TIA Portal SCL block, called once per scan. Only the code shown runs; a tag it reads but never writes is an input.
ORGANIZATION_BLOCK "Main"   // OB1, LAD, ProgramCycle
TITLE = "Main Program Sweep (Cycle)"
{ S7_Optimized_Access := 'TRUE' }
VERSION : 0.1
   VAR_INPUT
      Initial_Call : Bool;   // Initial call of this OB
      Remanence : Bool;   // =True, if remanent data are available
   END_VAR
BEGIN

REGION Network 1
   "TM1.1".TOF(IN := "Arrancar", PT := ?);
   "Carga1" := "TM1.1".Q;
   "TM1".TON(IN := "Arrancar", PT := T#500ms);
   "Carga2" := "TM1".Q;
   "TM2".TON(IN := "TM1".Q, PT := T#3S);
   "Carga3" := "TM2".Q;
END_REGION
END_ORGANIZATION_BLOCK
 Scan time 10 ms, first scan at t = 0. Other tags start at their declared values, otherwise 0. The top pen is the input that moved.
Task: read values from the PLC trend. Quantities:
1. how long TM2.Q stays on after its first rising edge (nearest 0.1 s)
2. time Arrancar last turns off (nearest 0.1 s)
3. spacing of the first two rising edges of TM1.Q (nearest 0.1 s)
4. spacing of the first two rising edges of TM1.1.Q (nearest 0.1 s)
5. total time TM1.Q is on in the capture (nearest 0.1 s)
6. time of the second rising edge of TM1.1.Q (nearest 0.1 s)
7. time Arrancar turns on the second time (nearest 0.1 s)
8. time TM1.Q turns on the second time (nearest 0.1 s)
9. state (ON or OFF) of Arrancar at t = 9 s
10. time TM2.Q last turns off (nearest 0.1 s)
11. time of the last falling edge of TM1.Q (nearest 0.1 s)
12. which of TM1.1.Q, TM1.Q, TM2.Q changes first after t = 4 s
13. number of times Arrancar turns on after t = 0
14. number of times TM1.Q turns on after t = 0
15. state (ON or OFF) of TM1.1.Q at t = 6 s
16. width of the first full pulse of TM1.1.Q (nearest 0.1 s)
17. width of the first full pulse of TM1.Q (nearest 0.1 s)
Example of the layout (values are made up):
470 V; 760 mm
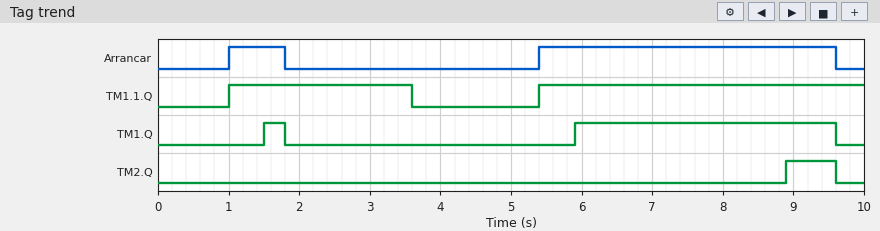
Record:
0.7 s; 9.6 s; 4.4 s; 4.4 s; 4.0 s; 5.4 s; 5.4 s; 5.9 s; ON; 9.6 s; 9.6 s; TM1.1.Q; 2; 2; ON; 2.6 s; 0.3 s
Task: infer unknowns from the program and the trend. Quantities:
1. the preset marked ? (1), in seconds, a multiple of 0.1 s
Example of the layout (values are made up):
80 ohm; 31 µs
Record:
1.8 s
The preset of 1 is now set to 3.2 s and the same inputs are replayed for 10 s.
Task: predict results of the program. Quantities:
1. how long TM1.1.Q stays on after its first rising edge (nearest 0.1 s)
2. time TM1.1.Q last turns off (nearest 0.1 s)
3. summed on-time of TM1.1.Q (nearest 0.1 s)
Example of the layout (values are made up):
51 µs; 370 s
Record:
4.0 s; 5.0 s; 8.6 s
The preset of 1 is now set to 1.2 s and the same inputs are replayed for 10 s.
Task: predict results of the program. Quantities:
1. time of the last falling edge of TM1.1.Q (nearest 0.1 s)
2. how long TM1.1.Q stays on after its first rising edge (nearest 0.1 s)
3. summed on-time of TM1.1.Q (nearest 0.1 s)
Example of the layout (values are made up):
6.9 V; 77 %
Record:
3.0 s; 2.0 s; 6.6 s
